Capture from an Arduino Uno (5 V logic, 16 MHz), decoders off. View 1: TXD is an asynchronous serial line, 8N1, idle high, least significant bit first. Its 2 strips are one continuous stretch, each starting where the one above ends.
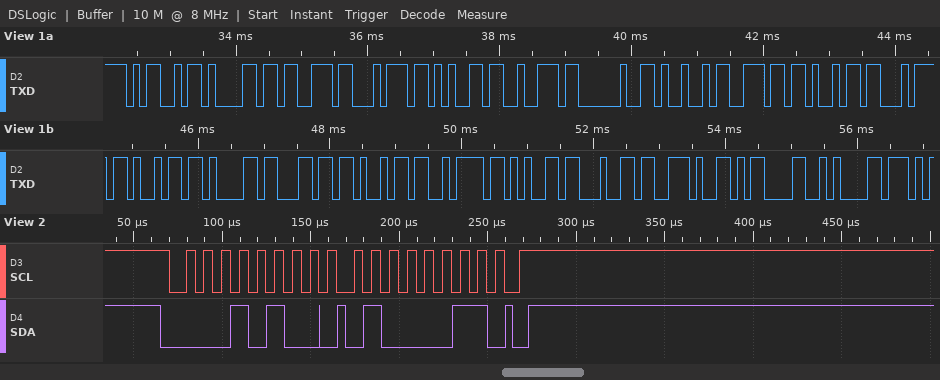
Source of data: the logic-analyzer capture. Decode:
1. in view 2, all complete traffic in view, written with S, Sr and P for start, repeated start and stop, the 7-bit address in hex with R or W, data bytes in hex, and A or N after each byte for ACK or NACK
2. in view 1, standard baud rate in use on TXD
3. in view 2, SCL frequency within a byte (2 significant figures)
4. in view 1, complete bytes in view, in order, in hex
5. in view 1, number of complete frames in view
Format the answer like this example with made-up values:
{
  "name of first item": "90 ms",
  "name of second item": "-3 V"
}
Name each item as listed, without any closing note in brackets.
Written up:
{
  "in view 2, all complete traffic in view, written with S, Sr and P for start, repeated start and stop, the 7-bit address in hex with R or W, data bytes in hex, and A or N after each byte for ACK or NACK": "S 0AW A 43 A P",
  "in view 1, standard baud rate in use on TXD": "9600 baud",
  "in view 2, SCL frequency within a byte": "100 kHz",
  "in view 1, complete bytes in view, in order, in hex": "4D 61 73 74 65 72 20 49 6E 69 74 69 61 6C 69 7A 65 64 2E 0D 0A",
  "in view 1, number of complete frames in view": "21"
}
